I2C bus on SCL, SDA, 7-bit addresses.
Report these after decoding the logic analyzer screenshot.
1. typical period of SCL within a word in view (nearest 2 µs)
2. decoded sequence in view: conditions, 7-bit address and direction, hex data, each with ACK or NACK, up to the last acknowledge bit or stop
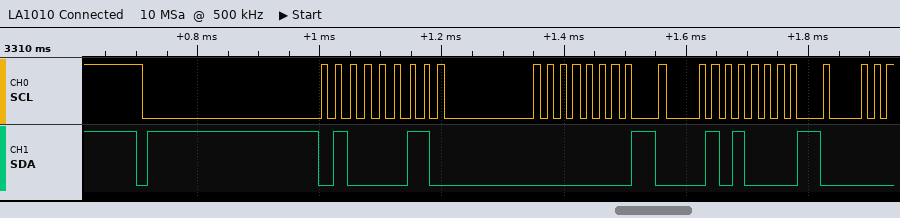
22 µs
start, address 21 read ACK, 00 ACK, 50 ACK
